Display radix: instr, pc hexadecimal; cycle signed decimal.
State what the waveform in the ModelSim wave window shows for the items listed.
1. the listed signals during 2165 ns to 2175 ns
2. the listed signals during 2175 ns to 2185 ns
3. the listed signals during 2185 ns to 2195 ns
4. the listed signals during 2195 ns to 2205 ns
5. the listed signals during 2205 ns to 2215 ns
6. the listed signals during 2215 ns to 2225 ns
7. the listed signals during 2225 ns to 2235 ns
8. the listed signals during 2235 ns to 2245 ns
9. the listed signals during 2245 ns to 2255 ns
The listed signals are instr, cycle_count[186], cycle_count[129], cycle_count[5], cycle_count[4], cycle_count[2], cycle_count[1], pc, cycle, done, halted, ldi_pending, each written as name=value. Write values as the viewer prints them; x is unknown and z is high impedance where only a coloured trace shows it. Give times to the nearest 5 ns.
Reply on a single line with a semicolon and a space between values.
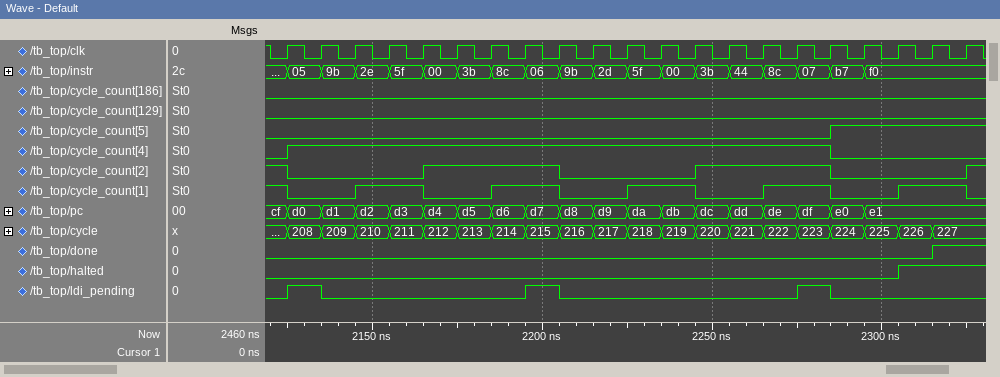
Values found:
instr=00, cycle_count[186]=0, cycle_count[129]=0, cycle_count[5]=0, cycle_count[4]=1, cycle_count[2]=1, cycle_count[1]=0, pc=d4, cycle=212, done=0, halted=0, ldi_pending=0; instr=3b, cycle_count[186]=0, cycle_count[129]=0, cycle_count[5]=0, cycle_count[4]=1, cycle_count[2]=1, cycle_count[1]=0, pc=d5, cycle=213, done=0, halted=0, ldi_pending=0; instr=8c, cycle_count[186]=0, cycle_count[129]=0, cycle_count[5]=0, cycle_count[4]=1, cycle_count[2]=1, cycle_count[1]=1, pc=d6, cycle=214, done=0, halted=0, ldi_pending=0; instr=06, cycle_count[186]=0, cycle_count[129]=0, cycle_count[5]=0, cycle_count[4]=1, cycle_count[2]=1, cycle_count[1]=1, pc=d7, cycle=215, done=0, halted=0, ldi_pending=1; instr=9b, cycle_count[186]=0, cycle_count[129]=0, cycle_count[5]=0, cycle_count[4]=1, cycle_count[2]=0, cycle_count[1]=0, pc=d8, cycle=216, done=0, halted=0, ldi_pending=0; instr=2d, cycle_count[186]=0, cycle_count[129]=0, cycle_count[5]=0, cycle_count[4]=1, cycle_count[2]=0, cycle_count[1]=0, pc=d9, cycle=217, done=0, halted=0, ldi_pending=0; instr=5f, cycle_count[186]=0, cycle_count[129]=0, cycle_count[5]=0, cycle_count[4]=1, cycle_count[2]=0, cycle_count[1]=1, pc=da, cycle=218, done=0, halted=0, ldi_pending=0; instr=00, cycle_count[186]=0, cycle_count[129]=0, cycle_count[5]=0, cycle_count[4]=1, cycle_count[2]=0, cycle_count[1]=1, pc=db, cycle=219, done=0, halted=0, ldi_pending=0; instr=3b, cycle_count[186]=0, cycle_count[129]=0, cycle_count[5]=0, cycle_count[4]=1, cycle_count[2]=1, cycle_count[1]=0, pc=dc, cycle=220, done=0, halted=0, ldi_pending=0
